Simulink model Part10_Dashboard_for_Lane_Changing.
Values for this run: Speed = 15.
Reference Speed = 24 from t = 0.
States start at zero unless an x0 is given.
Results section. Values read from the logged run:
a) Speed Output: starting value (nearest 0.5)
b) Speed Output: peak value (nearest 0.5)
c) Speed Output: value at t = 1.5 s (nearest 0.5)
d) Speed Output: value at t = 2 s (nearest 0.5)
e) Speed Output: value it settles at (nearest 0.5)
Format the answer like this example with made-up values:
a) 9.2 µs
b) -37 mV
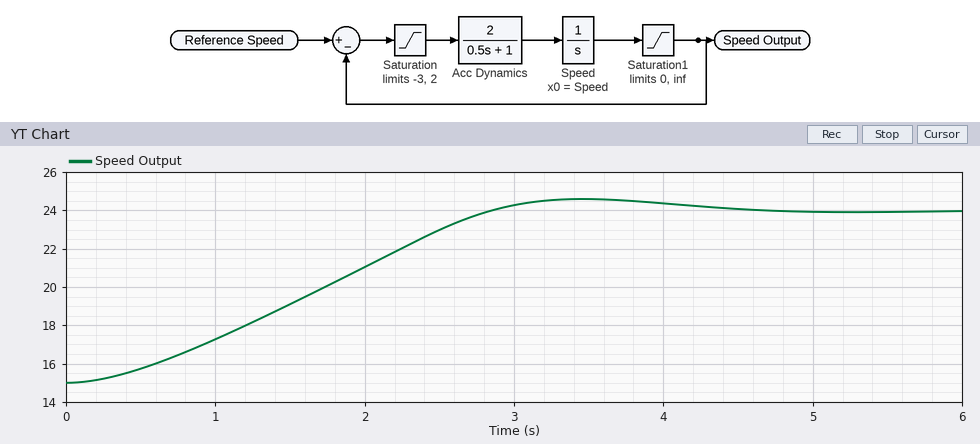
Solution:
a) 15.0
b) 24.5
c) 19.0
d) 21.0
e) 24.0
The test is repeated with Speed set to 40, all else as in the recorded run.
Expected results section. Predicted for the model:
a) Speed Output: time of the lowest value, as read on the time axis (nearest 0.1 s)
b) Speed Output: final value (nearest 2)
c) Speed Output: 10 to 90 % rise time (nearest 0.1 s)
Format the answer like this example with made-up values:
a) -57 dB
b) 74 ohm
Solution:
a) 3.9 s
b) 24
c) 2.3 s
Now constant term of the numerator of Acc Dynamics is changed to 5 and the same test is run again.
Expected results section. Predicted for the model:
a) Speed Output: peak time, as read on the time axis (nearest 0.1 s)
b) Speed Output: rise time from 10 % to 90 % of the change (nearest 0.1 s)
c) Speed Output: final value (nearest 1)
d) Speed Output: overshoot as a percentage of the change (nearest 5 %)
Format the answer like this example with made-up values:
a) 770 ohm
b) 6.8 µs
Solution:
a) 1.8 s
b) 0.9 s
c) 24
d) 15 %
